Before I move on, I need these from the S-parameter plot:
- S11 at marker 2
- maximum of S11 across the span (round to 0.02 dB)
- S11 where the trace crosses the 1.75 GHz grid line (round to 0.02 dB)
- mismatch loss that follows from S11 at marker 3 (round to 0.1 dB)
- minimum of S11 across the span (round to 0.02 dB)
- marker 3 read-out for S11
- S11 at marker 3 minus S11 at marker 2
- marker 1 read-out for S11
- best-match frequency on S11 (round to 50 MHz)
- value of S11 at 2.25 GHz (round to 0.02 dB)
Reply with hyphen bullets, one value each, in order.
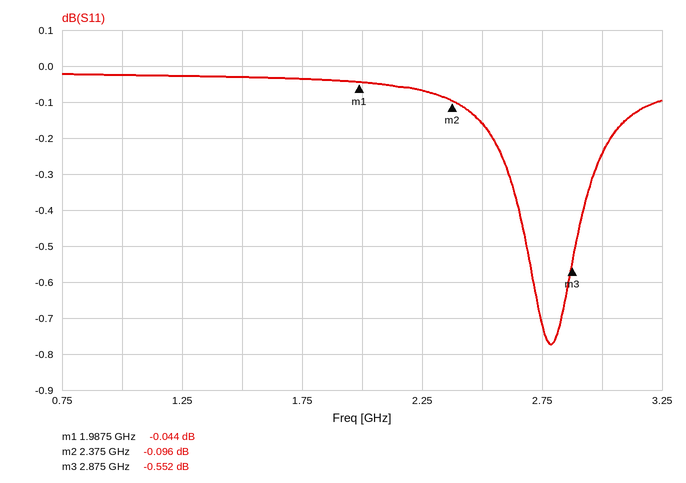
- -0.096 dB
- -0.02 dB
- -0.04 dB
- 9.2 dB
- -0.78 dB
- -0.552 dB
- -0.456 dB
- -0.044 dB
- 2.80 GHz
- -0.06 dB
